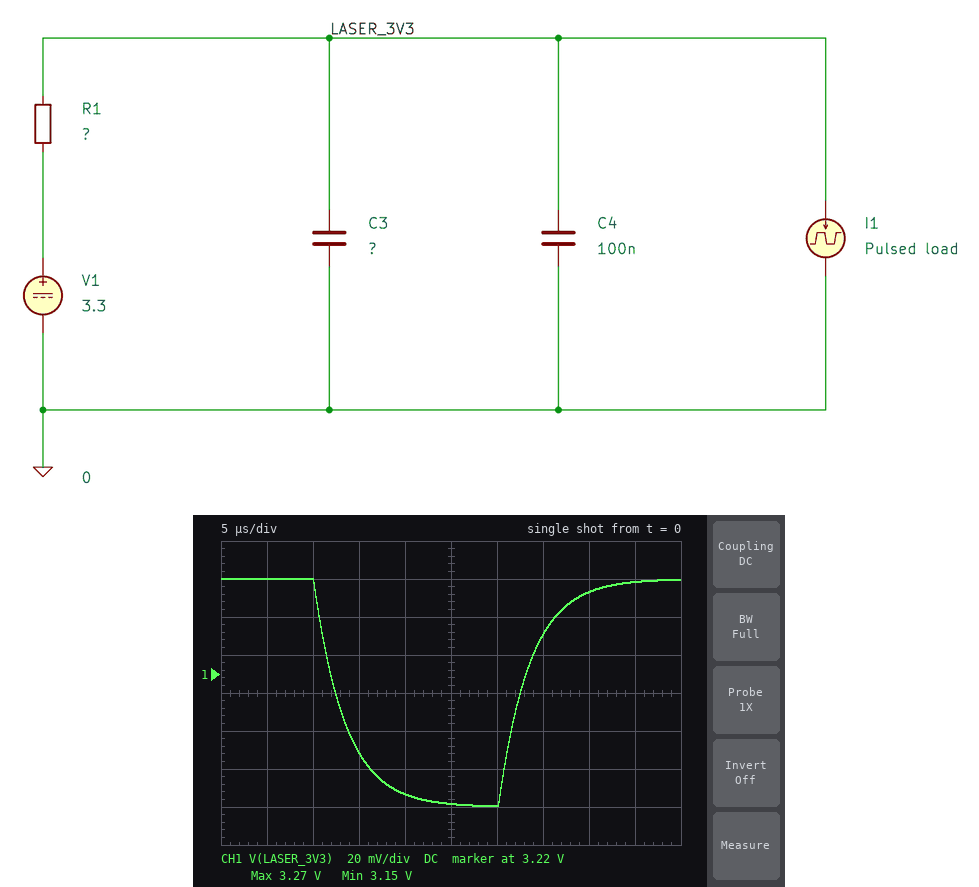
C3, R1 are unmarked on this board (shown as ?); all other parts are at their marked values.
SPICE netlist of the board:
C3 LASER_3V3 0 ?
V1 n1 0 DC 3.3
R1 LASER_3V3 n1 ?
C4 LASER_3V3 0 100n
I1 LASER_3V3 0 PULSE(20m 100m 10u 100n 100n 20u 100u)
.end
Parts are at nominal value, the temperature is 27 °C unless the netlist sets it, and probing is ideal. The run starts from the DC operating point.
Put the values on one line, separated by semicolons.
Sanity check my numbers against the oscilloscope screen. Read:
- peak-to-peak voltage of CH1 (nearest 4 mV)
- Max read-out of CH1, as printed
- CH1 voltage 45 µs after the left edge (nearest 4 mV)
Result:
120 mV; 3.27 V; 3.268 V
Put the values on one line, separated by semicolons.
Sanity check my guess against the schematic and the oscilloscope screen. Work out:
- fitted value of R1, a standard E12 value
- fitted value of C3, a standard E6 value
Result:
1.5 Ω; 2.2 µF
